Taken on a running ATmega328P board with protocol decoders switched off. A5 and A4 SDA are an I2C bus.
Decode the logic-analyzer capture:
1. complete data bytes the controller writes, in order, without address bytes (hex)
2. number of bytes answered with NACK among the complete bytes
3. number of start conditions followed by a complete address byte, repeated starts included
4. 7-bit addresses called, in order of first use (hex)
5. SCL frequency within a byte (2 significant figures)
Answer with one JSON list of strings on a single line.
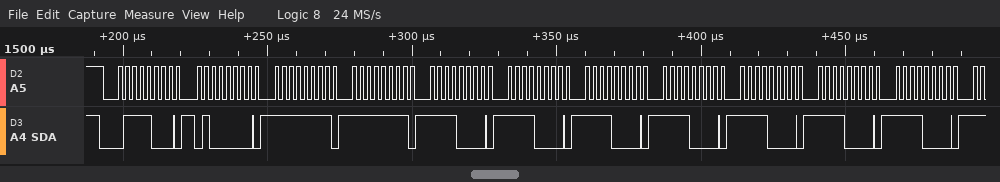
["40 FF FF F0 F0 F0 F0 F0 F0 F0", "0", "1", "0x3C", "400 kHz"]
